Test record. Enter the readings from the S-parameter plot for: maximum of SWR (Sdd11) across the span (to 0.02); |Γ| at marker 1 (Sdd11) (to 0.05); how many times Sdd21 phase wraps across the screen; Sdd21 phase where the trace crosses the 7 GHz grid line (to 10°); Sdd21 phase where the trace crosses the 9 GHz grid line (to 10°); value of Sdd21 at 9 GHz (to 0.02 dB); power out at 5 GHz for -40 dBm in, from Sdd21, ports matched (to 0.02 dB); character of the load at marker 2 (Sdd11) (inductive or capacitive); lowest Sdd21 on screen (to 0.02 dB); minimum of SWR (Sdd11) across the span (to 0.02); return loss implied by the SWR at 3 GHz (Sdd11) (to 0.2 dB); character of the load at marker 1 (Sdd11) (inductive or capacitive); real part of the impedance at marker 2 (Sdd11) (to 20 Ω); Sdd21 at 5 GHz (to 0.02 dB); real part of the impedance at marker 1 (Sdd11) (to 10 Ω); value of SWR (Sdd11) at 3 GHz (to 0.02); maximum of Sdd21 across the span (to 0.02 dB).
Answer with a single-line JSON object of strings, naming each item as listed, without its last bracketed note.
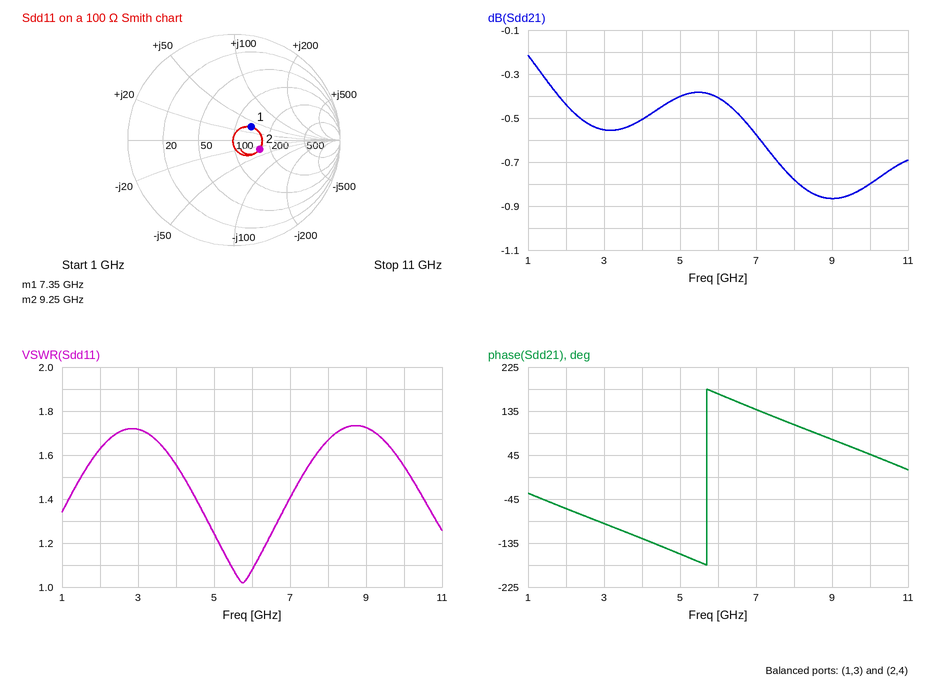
{"maximum of SWR (Sdd11) across the span": "1.74", "|Γ| at marker 1 (Sdd11)": "0.20", "how many times Sdd21 phase wraps across the screen": "1", "Sdd21 phase where the trace crosses the 7 GHz grid line": "140°", "Sdd21 phase where the trace crosses the 9 GHz grid line": "80°", "value of Sdd21 at 9 GHz": "-0.86 dB", "power out at 5 GHz for -40 dBm in, from Sdd21, ports matched": "-40.40 dBm", "character of the load at marker 2 (Sdd11)": "capacitive", "lowest Sdd21 on screen": "-0.86 dB", "minimum of SWR (Sdd11) across the span": "1.02", "return loss implied by the SWR at 3 GHz (Sdd11)": "11.6 dB", "character of the load at marker 1 (Sdd11)": "inductive", "real part of the impedance at marker 2 (Sdd11)": "160 Ω", "Sdd21 at 5 GHz": "-0.40 dB", "real part of the impedance at marker 1 (Sdd11)": "130 Ω", "value of SWR (Sdd11) at 3 GHz": "1.72", "maximum of Sdd21 across the span": "-0.22 dB"}
